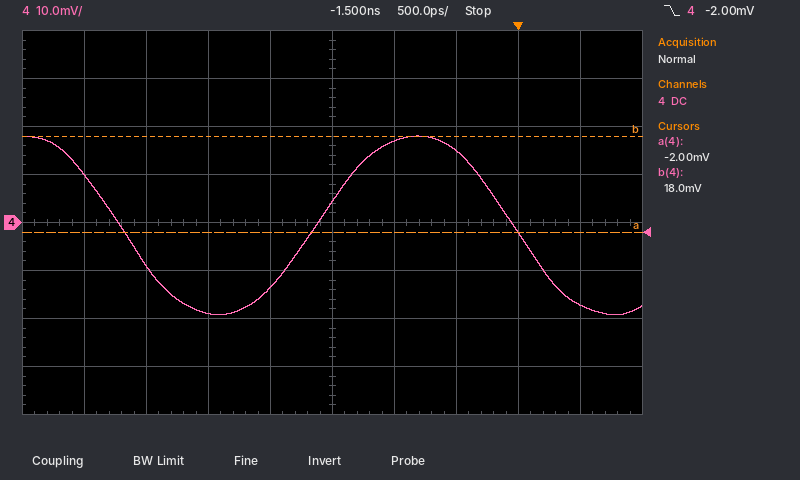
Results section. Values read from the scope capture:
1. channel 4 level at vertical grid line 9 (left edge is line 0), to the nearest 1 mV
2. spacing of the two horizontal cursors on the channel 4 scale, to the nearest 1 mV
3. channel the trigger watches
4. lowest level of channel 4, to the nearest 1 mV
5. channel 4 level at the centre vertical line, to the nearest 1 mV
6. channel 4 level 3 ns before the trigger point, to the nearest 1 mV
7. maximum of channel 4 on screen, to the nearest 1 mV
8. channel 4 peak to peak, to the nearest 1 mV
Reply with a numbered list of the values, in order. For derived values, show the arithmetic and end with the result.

1. -17 mV
2. 20 mV
3. channel 4
4. -19 mV
5. 4 mV
6. -9 mV
7. 18 mV
8. 18 mV − (-19 mV) = 37 mV
